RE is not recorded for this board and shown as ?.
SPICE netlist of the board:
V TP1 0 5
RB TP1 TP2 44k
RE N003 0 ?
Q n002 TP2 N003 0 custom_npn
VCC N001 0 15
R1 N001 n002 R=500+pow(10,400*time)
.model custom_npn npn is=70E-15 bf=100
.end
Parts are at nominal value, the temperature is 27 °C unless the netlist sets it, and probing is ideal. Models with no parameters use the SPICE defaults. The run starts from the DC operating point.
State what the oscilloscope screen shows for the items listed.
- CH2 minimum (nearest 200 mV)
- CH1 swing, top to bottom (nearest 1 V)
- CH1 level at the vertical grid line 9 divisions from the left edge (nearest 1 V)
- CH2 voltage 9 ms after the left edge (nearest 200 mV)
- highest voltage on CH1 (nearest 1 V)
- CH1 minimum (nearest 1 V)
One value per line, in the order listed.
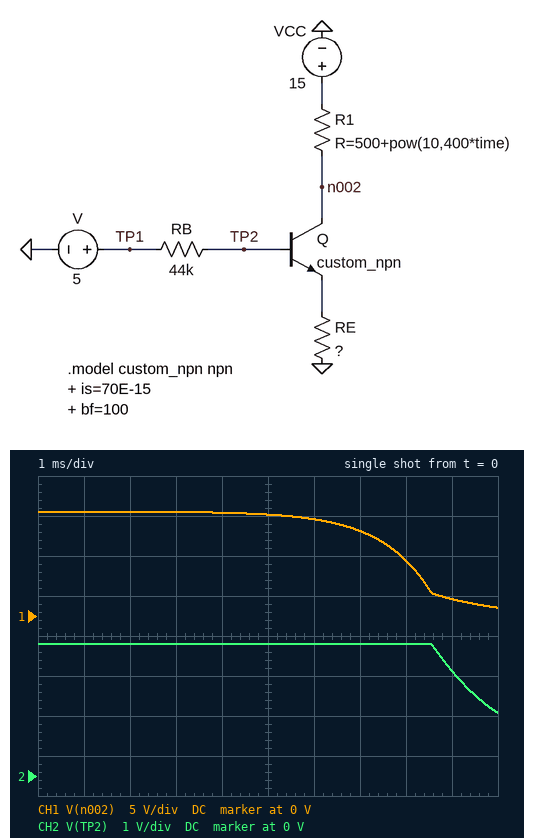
1.6 V
12 V
2 V
2.6 V
13 V
1 V
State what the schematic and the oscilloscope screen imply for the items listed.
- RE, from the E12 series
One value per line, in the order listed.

680 Ω
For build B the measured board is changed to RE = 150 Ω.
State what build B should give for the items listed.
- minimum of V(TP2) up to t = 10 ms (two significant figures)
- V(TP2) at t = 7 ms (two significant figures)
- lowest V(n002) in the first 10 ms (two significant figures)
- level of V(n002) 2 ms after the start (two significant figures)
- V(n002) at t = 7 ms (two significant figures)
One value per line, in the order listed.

840 mV
1.8 V
300 mV
11 V
6.7 V
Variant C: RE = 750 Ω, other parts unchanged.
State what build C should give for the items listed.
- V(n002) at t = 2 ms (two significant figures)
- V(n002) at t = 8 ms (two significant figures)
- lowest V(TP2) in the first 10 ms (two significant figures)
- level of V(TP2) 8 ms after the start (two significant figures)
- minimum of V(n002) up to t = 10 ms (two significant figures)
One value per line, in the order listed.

13 V
7.4 V
1.7 V
3.4 V
1.1 V
